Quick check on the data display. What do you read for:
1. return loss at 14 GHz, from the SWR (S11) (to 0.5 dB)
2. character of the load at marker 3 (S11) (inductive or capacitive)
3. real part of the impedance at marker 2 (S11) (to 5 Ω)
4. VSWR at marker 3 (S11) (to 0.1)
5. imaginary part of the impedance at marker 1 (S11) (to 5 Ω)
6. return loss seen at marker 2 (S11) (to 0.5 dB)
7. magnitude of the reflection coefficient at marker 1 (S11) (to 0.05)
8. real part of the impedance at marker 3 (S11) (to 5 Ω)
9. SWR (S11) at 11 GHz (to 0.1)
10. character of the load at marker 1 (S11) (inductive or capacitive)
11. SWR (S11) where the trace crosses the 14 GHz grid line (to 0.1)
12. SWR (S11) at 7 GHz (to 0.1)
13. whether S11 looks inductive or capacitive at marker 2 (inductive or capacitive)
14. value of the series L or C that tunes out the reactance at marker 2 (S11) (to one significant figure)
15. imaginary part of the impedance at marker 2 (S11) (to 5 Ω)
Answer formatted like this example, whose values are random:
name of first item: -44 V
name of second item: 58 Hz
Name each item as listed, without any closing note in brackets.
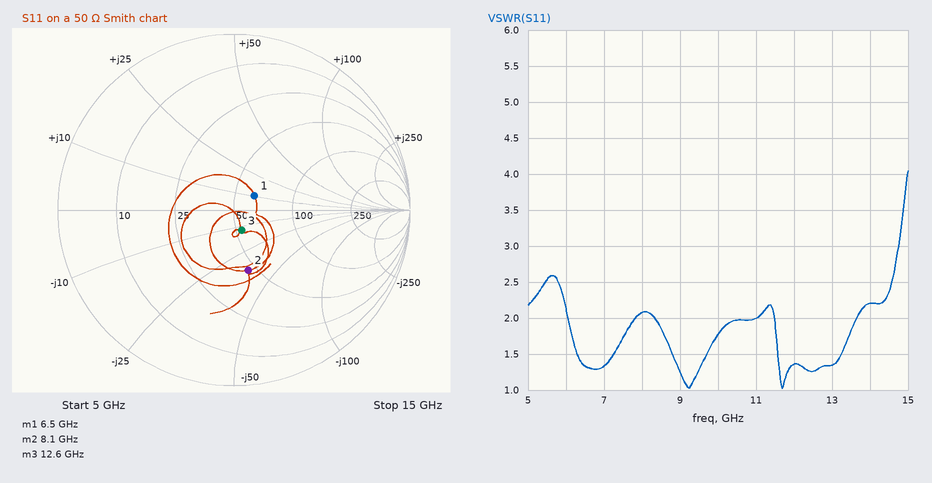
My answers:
return loss at 14 GHz, from the SWR (S11): 8.5 dB
character of the load at marker 3 (S11): capacitive
real part of the impedance at marker 2 (S11): 45 Ω
VSWR at marker 3 (S11): 1.3
imaginary part of the impedance at marker 1 (S11): +10 Ω
return loss seen at marker 2 (S11): 9.0 dB
magnitude of the reflection coefficient at marker 1 (S11): 0.15
real part of the impedance at marker 3 (S11): 55 Ω
SWR (S11) at 11 GHz: 2.0
character of the load at marker 1 (S11): inductive
SWR (S11) where the trace crosses the 14 GHz grid line: 2.2
SWR (S11) at 7 GHz: 1.3
whether S11 looks inductive or capacitive at marker 2: capacitive
value of the series L or C that tunes out the reactance at marker 2 (S11): 700 pH
imaginary part of the impedance at marker 2 (S11): -35 Ω
